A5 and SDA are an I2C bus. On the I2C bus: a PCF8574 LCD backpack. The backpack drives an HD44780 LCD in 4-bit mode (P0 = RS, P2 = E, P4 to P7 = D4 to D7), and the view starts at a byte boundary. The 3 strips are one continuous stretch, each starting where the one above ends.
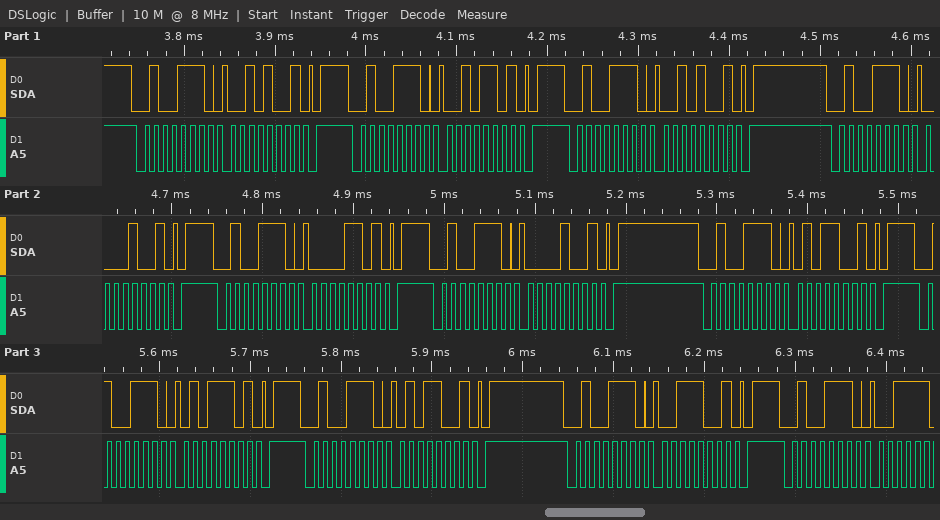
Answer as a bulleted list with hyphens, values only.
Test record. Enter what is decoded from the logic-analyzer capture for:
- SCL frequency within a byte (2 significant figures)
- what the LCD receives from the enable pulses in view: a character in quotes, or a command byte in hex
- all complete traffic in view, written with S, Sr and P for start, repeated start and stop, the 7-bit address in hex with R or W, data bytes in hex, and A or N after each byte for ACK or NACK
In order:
- 100 kHz
- ' '
- S 27W A 29 A P S 27W A 2D A P S 27W A 29 A P S 27W A 09 A P S 27W A 0D A P S 27W A 09 A P S 27W A 59 A P S 27W A 5D A P S 27W A 59 A P S 27W A 39 A P S 27W A
